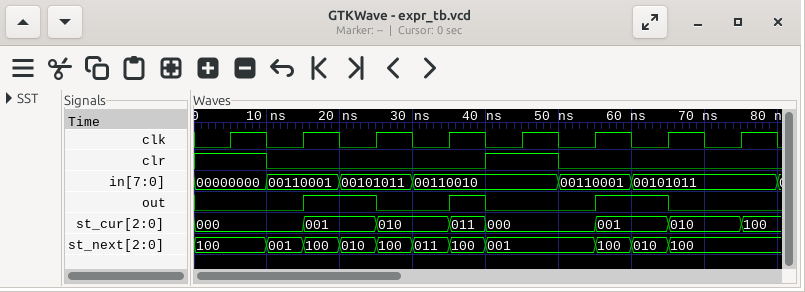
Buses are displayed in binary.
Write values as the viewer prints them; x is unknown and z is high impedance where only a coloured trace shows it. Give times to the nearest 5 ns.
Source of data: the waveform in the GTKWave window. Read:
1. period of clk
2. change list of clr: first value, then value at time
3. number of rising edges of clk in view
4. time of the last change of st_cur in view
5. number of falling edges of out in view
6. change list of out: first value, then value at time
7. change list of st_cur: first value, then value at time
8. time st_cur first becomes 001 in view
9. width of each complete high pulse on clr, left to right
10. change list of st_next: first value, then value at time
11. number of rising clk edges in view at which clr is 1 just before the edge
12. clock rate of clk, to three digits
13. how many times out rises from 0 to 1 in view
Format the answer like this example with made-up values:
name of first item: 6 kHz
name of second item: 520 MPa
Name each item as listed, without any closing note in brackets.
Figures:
period of clk: 10 ns
change list of clr: first value, then value at time: 1, 0 at 10 ns, 1 at 40 ns, 0 at 50 ns
number of rising edges of clk in view: 8
time of the last change of st_cur in view: 75 ns
number of falling edges of out in view: 3
change list of out: first value, then value at time: 0, 1 at 15 ns, 0 at 25 ns, 1 at 35 ns, 0 at 40 ns, 1 at 55 ns, 0 at 65 ns
change list of st_cur: first value, then value at time: 000, 001 at 15 ns, 010 at 25 ns, 011 at 35 ns, 000 at 40 ns, 001 at 55 ns, 010 at 65 ns, 100 at 75 ns
time st_cur first becomes 001 in view: 15 ns
width of each complete high pulse on clr, left to right: 10 ns
change list of st_next: first value, then value at time: 100, 001 at 10 ns, 100 at 15 ns, 010 at 20 ns, 100 at 25 ns, 011 at 30 ns, 100 at 35 ns, 001 at 40 ns, 100 at 55 ns, 010 at 60 ns, 100 at 65 ns
number of rising clk edges in view at which clr is 1 just before the edge: 2
clock rate of clk, to three digits: 100 MHz
how many times out rises from 0 to 1 in view: 3
